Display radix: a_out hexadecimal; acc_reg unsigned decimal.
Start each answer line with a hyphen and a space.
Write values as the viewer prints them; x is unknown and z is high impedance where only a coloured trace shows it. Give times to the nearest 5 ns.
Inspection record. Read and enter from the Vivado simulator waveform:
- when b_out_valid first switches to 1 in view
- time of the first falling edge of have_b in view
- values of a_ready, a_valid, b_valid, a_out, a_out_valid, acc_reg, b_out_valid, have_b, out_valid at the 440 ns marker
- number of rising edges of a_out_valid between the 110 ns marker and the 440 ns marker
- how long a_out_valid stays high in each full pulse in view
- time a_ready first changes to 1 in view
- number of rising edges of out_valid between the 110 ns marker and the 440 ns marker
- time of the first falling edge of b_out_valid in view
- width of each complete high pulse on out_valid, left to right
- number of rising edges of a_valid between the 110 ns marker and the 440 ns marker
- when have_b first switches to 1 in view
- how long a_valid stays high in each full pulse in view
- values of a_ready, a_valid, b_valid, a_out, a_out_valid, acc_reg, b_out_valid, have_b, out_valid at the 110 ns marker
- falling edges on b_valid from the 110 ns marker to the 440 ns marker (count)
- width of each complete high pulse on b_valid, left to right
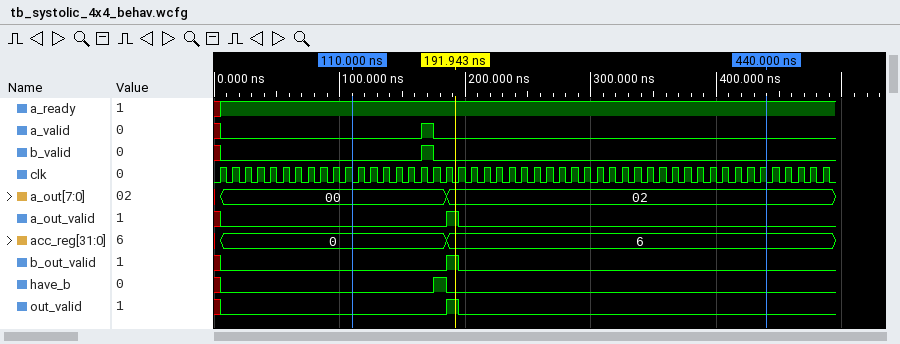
- 185 ns
- 185 ns
- a_ready=1, a_valid=0, b_valid=0, a_out=02, a_out_valid=0, acc_reg=6, b_out_valid=0, have_b=0, out_valid=0
- 1
- 10 ns
- 5 ns
- 1
- 195 ns
- 10 ns
- 1
- 175 ns
- 10 ns
- a_ready=1, a_valid=0, b_valid=0, a_out=00, a_out_valid=0, acc_reg=0, b_out_valid=0, have_b=0, out_valid=0
- 1
- 10 ns
